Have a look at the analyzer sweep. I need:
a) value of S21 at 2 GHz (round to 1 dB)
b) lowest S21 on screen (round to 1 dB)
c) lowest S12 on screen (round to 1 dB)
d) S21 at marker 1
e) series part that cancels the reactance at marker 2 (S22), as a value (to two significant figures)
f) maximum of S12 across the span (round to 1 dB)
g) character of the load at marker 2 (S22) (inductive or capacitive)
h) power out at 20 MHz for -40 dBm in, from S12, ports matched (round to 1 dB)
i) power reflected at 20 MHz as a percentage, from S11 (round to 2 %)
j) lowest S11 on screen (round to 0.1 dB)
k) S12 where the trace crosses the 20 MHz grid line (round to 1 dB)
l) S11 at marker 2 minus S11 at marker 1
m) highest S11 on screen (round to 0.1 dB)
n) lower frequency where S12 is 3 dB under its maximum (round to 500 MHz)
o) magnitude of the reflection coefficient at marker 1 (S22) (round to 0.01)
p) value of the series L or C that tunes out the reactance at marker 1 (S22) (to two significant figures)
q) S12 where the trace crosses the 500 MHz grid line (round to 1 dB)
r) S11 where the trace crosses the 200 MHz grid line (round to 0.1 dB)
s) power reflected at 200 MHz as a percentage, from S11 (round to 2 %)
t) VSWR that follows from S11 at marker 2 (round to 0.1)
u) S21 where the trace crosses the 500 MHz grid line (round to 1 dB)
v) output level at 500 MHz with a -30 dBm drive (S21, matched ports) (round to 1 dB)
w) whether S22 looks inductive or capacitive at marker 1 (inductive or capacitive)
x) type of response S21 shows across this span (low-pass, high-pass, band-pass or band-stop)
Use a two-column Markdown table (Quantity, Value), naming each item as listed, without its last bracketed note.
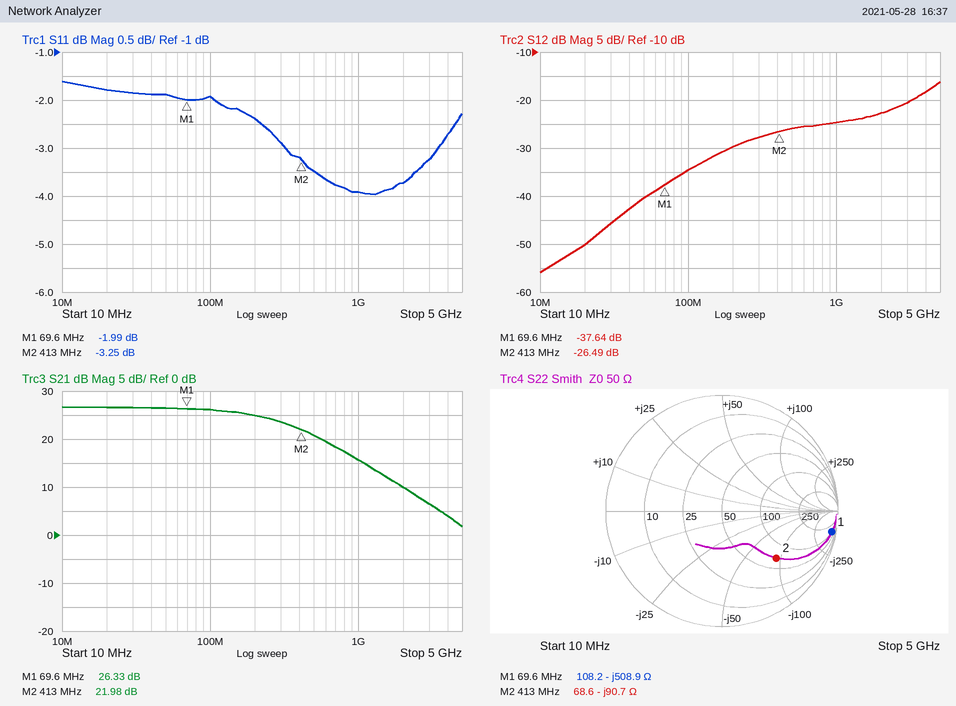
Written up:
| Quantity | Value |
|---|---|
| value of S21 at 2 GHz | 10 dB |
| lowest S21 on screen | 2 dB |
| lowest S12 on screen | -56 dB |
| S21 at marker 1 | 26.33 dB |
| series part that cancels the reactance at marker 2 (S22), as a value | 35 nH |
| maximum of S12 across the span | -16 dB |
| character of the load at marker 2 (S22) | capacitive |
| power out at 20 MHz for -40 dBm in, from S12, ports matched | -90 dBm |
| power reflected at 20 MHz as a percentage, from S11 | 66 % |
| lowest S11 on screen | -4.0 dB |
| S12 where the trace crosses the 20 MHz grid line | -50 dB |
| S11 at marker 2 minus S11 at marker 1 | -1.26 dB |
| highest S11 on screen | -1.6 dB |
| lower frequency where S12 is 3 dB under its maximum | 3.5 GHz |
| magnitude of the reflection coefficient at marker 1 (S22) | 0.96 |
| value of the series L or C that tunes out the reactance at marker 1 (S22) | 1.2 µH |
| S12 where the trace crosses the 500 MHz grid line | -26 dB |
| S11 where the trace crosses the 200 MHz grid line | -2.4 dB |
| power reflected at 200 MHz as a percentage, from S11 | 58 % |
| VSWR that follows from S11 at marker 2 | 5.4 |
| S21 where the trace crosses the 500 MHz grid line | 21 dB |
| output level at 500 MHz with a -30 dBm drive (S21, matched ports) | -9 dBm |
| whether S22 looks inductive or capacitive at marker 1 | capacitive |
| type of response S21 shows across this span | low-pass |
